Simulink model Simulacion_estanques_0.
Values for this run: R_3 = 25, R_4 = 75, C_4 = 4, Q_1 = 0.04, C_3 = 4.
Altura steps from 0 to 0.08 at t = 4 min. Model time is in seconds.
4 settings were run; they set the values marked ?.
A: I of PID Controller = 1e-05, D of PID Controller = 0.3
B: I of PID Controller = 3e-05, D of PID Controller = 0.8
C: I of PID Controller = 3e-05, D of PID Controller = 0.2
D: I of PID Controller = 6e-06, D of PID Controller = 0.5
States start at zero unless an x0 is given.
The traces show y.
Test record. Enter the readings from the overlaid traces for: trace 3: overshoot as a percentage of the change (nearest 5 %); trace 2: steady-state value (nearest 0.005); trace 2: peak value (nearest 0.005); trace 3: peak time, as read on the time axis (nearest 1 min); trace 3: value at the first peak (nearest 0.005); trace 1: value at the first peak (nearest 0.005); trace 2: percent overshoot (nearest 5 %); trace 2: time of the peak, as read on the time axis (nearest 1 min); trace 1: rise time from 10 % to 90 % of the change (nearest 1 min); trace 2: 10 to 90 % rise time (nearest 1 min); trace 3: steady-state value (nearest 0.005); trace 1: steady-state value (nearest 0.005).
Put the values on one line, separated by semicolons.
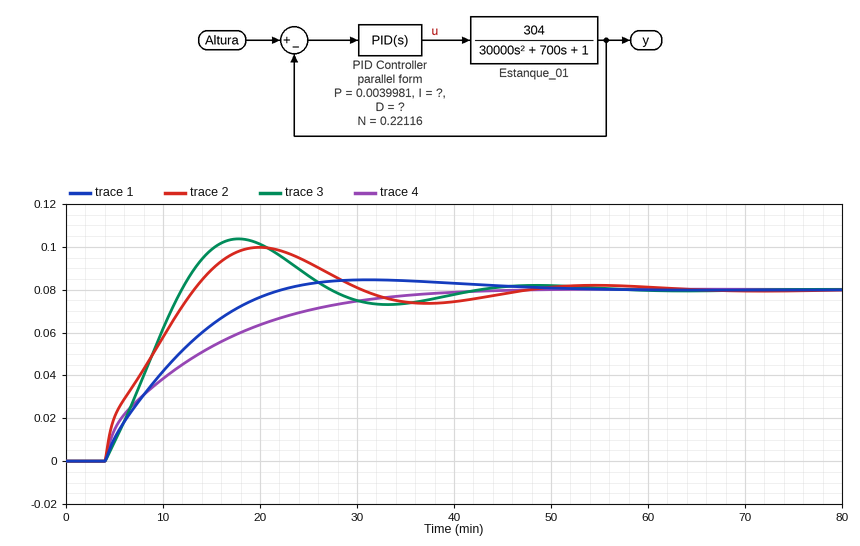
30 %; 0.080; 0.100; 18 min; 0.105; 0.085; 25 %; 20 min; 13 min; 8 min; 0.080; 0.080
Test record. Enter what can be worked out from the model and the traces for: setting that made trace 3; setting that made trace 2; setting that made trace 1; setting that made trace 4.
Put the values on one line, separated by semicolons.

C; B; A; D
